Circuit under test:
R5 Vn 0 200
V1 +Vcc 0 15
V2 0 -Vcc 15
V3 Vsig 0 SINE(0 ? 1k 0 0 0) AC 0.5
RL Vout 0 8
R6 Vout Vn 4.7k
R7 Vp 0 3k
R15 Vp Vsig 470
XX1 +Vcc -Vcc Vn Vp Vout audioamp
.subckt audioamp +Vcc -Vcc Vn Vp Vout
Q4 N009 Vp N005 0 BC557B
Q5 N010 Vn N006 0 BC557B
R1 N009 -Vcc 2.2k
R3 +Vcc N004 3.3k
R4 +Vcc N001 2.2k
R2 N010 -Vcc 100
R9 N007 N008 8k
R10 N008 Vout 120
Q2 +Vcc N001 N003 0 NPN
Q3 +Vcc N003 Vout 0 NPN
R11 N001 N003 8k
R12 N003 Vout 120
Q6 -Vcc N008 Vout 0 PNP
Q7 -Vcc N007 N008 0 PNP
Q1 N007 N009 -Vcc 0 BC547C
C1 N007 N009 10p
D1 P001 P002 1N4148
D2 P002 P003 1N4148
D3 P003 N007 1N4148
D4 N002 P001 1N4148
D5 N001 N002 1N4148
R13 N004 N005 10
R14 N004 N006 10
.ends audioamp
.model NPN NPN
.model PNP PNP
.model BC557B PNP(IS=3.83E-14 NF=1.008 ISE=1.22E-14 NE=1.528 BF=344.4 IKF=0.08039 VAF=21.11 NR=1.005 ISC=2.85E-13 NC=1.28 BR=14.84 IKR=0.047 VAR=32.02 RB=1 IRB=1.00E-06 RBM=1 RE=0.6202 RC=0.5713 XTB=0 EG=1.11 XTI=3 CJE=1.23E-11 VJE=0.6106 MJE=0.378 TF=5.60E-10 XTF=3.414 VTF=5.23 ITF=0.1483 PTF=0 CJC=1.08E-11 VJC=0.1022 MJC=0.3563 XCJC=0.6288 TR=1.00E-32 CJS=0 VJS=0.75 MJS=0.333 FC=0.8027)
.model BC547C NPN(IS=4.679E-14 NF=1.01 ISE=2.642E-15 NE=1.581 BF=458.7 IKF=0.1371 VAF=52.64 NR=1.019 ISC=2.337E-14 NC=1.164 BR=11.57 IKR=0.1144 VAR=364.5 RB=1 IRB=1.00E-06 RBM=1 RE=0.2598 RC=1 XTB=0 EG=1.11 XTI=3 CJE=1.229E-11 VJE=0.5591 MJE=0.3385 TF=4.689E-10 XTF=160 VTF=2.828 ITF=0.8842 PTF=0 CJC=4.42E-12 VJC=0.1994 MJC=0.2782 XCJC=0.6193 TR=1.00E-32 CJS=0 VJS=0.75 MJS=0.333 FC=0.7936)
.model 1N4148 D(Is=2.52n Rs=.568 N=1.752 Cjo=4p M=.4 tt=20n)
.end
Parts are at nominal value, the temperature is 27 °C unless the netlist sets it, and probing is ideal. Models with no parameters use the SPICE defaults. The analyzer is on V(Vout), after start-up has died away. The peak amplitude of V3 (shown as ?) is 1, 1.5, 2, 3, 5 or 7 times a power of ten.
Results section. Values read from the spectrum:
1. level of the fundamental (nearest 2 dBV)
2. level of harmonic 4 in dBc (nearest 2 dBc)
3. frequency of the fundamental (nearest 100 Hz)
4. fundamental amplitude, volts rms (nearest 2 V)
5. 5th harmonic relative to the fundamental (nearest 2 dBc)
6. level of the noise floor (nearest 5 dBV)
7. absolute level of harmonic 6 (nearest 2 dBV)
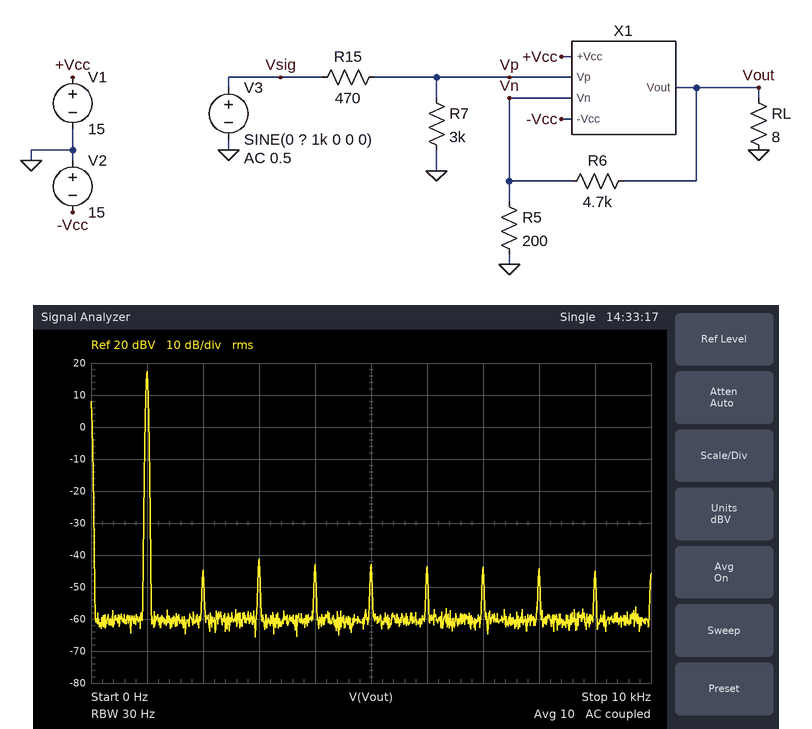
18 dBV
-60 dBc
1.0 kHz
8 V
-60 dBc
-60 dBV
-44 dBV
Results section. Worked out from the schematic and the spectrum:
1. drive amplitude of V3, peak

500 mV
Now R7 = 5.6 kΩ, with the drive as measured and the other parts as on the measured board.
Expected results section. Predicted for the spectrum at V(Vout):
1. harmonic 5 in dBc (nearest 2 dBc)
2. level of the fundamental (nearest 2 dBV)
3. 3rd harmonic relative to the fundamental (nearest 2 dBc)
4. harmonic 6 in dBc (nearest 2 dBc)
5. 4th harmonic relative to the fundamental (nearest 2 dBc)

-42 dBc
18 dBV
-40 dBc
-44 dBc
-40 dBc
